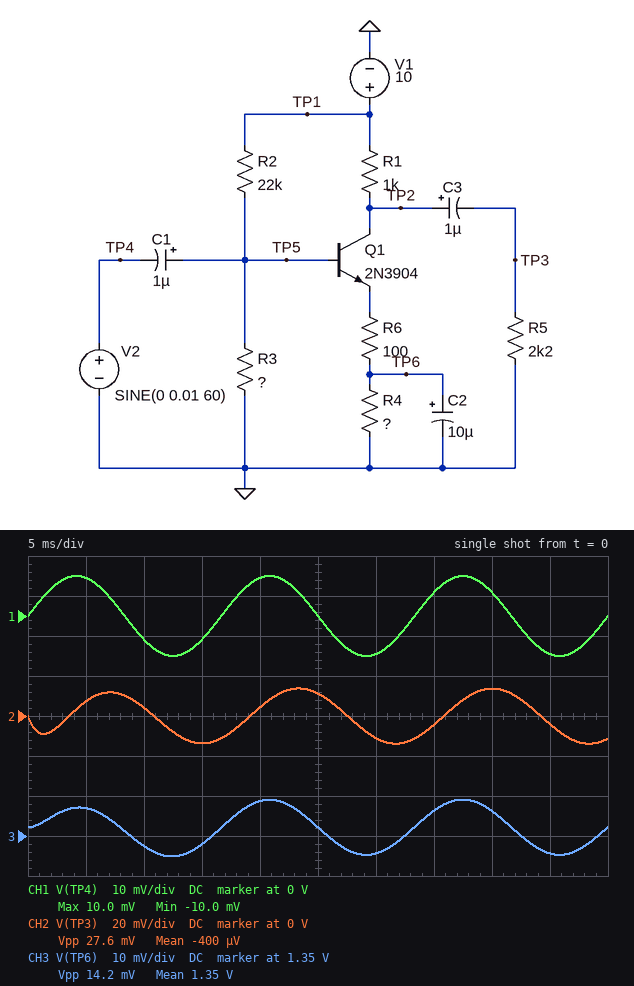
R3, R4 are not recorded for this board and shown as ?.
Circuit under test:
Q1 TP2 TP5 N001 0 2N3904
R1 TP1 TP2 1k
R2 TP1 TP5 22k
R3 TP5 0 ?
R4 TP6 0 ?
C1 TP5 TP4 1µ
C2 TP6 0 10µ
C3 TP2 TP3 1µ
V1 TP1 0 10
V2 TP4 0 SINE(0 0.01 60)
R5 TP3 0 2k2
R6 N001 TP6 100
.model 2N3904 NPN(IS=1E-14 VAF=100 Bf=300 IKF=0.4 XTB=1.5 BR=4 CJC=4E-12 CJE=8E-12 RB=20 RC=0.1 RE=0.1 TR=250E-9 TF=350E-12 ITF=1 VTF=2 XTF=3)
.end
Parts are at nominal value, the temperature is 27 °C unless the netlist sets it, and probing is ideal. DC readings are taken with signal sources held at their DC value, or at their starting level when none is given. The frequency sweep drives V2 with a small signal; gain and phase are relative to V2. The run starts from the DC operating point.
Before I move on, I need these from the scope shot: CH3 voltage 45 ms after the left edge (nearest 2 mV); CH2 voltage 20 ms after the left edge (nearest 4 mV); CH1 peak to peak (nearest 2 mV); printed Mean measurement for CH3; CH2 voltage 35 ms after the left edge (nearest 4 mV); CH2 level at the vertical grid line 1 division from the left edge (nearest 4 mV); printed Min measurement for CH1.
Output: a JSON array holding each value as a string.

["1.346 V", "4 mV", "20 mV", "1.35 V", "-4 mV", "8 mV", "-10.0 mV"]
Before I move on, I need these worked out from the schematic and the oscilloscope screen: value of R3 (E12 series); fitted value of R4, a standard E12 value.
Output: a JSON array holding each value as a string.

["5.6 kΩ", "3.3 kΩ"]
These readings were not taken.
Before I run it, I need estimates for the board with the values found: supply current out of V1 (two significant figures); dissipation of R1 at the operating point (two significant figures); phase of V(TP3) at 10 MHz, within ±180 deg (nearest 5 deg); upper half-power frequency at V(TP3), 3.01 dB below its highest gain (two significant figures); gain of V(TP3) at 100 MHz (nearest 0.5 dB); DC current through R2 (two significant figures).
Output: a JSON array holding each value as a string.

["770 µA", "170 µW", "170 deg", "100 MHz", "9.5 dB", "360 µA"]
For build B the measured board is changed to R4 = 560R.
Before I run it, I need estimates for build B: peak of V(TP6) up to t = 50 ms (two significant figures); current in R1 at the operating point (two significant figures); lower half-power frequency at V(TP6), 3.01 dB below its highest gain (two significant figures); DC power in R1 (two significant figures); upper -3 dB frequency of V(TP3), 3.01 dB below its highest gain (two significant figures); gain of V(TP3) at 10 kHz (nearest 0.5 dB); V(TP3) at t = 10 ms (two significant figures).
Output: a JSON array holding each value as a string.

["1.1 V", "2.0 mA", "26 Hz", "4.0 mW", "95 MHz", "15.5 dB", "6.4 mV"]
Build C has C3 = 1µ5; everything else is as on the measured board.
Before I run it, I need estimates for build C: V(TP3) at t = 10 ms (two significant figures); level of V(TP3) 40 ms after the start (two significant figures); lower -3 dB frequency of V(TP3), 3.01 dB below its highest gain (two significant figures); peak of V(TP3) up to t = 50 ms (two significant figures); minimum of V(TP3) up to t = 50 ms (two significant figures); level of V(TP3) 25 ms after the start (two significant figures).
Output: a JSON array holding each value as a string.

["6.9 mV", "15 mV", "120 Hz", "16 mV", "-16 mV", "14 mV"]
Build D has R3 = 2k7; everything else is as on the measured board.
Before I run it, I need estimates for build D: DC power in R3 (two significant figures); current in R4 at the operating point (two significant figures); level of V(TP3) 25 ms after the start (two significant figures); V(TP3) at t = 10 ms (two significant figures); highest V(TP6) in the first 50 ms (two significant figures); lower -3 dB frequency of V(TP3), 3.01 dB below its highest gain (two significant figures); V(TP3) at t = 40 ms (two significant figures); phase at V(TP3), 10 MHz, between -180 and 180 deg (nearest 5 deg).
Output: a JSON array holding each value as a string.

["440 µW", "140 µA", "6.7 mV", "2.3 mV", "480 mV", "120 Hz", "8.6 mV", "170 deg"]
